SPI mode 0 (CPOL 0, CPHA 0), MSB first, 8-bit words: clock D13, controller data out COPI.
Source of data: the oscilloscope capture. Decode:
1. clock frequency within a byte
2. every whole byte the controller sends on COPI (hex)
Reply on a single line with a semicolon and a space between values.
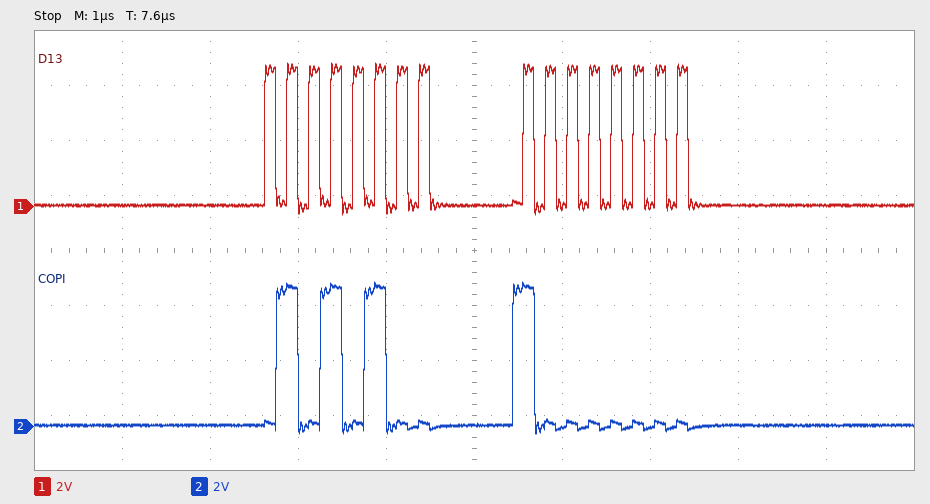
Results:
4 MHz; 54 80
